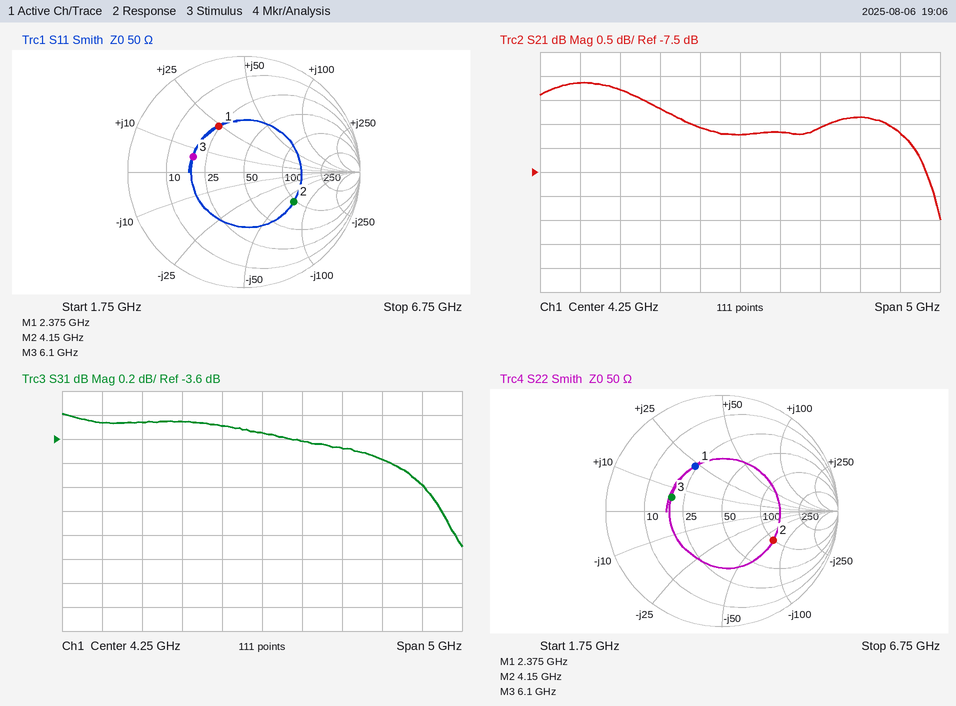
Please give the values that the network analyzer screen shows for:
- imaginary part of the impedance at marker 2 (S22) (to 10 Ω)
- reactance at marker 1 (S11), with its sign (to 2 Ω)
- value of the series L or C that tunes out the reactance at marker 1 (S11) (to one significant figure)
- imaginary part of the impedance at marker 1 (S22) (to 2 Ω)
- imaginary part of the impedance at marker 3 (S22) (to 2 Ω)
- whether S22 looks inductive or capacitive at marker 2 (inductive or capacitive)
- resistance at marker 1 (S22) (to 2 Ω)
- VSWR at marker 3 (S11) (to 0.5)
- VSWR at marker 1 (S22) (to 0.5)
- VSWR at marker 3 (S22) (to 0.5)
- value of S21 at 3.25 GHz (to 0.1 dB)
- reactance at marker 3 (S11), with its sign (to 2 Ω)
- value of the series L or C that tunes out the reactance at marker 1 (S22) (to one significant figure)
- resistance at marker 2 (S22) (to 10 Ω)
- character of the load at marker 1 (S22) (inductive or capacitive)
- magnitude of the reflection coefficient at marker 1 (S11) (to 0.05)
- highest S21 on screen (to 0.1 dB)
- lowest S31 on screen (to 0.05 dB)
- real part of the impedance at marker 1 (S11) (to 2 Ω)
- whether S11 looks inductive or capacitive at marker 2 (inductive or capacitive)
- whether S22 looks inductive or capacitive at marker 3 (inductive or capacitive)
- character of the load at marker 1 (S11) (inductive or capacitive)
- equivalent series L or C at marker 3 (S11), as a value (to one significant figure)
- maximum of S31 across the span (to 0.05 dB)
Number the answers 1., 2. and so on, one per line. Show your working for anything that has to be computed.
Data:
1. -70 Ω
2. +24 Ω
3. C = 1/(2π × 2.375 GHz × 24 Ω) ≈ 3 pF
4. +24 Ω
5. +6 Ω
6. capacitive
7. 24 Ω
8. 2.5
9. 2.5
10. 2.5
11. -6.2 dB
12. +6 Ω
13. C = 1/(2π × 2.375 GHz × 24 Ω) ≈ 3 pF
14. 100 Ω
15. inductive
16. 0.45
17. -5.6 dB
18. -4.50 dB
19. 24 Ω
20. capacitive
21. inductive
22. inductive
23. L = 6 Ω/(2π × 6.1 GHz) ≈ 157 pH, so 200 pH to one significant figure
24. -3.40 dB
